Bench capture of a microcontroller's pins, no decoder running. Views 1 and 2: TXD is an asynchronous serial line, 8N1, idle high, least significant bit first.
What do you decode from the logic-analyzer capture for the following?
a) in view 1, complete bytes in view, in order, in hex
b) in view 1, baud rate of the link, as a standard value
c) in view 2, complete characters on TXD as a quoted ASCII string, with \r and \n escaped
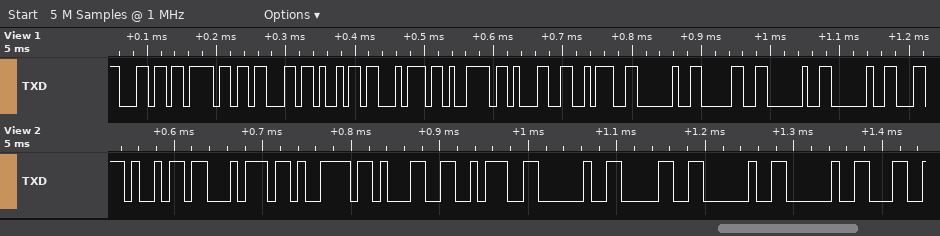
6C 6F 63 69 74 79 31 3A 20 30 20 20
115200 baud
"ity1: 0  "
